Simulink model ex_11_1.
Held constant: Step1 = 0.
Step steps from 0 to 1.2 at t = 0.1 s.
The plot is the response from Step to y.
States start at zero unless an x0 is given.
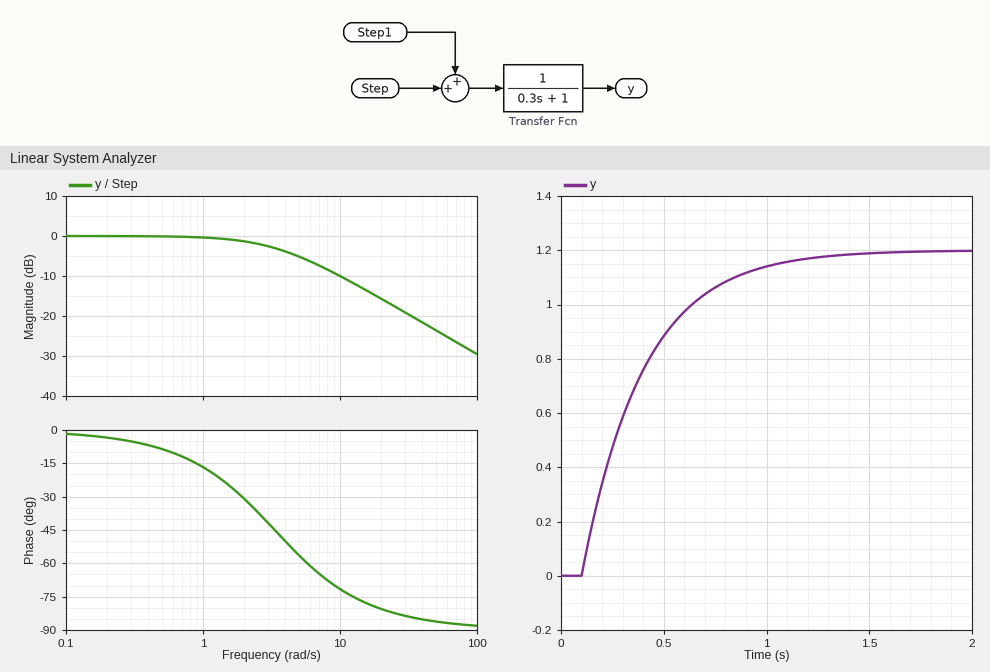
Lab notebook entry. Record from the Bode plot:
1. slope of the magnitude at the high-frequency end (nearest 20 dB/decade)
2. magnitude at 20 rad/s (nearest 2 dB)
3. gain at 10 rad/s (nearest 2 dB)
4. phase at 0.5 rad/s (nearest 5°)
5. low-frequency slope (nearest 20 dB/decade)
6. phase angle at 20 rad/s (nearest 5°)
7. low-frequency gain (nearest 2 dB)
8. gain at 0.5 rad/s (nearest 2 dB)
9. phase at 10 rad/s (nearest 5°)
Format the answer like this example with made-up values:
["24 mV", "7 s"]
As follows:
["-20 dB/decade", "-16 dB", "-10 dB", "-10°", "0 dB/decade", "-80°", "0 dB", "0 dB", "-70°"]
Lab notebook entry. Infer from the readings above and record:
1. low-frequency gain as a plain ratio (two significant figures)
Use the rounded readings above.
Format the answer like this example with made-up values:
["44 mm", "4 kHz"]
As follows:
["1.0"]
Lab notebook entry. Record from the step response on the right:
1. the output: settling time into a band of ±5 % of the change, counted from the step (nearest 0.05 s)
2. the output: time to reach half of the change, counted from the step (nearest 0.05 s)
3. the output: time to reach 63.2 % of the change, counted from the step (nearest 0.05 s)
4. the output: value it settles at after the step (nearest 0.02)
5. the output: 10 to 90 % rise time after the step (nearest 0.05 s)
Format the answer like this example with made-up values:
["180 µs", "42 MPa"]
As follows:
["0.90 s", "0.20 s", "0.30 s", "1.20", "0.65 s"]
